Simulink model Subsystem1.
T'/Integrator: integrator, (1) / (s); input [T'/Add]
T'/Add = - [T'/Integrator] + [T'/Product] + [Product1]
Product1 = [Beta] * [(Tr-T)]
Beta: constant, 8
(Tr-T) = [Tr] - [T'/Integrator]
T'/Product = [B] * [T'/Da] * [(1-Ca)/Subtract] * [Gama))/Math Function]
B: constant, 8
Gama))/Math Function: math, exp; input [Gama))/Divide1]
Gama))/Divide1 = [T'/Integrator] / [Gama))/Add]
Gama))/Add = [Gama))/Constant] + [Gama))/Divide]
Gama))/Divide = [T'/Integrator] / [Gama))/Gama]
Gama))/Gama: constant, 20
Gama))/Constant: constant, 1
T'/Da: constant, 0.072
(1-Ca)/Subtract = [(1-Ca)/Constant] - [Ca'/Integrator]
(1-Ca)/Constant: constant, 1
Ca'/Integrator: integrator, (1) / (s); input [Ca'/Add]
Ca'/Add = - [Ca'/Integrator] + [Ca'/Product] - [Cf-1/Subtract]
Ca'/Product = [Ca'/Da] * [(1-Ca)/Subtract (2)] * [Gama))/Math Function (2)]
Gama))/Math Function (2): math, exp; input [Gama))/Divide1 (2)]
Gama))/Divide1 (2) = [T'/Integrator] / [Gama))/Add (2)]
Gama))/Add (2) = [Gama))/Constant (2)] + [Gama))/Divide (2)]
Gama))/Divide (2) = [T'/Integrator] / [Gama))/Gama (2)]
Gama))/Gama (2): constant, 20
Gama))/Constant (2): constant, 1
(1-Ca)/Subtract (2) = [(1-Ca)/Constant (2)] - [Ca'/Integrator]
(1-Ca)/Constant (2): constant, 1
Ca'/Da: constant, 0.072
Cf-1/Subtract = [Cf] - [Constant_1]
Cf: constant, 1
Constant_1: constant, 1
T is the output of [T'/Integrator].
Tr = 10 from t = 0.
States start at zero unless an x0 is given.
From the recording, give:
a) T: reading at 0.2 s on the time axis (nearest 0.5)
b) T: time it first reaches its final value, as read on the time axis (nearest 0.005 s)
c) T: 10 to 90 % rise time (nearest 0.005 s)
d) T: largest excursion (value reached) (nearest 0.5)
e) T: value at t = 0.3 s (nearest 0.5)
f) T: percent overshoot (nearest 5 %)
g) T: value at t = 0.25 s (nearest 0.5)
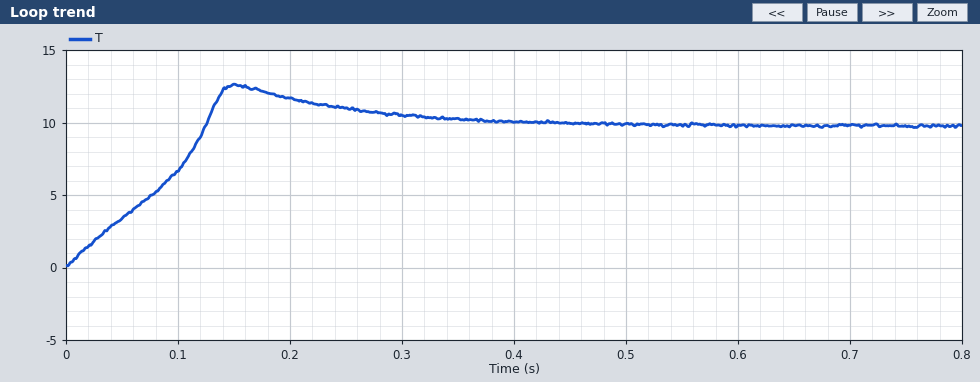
11.5
0.125 s
0.105 s
12.5
10.5
30 %
11.0
